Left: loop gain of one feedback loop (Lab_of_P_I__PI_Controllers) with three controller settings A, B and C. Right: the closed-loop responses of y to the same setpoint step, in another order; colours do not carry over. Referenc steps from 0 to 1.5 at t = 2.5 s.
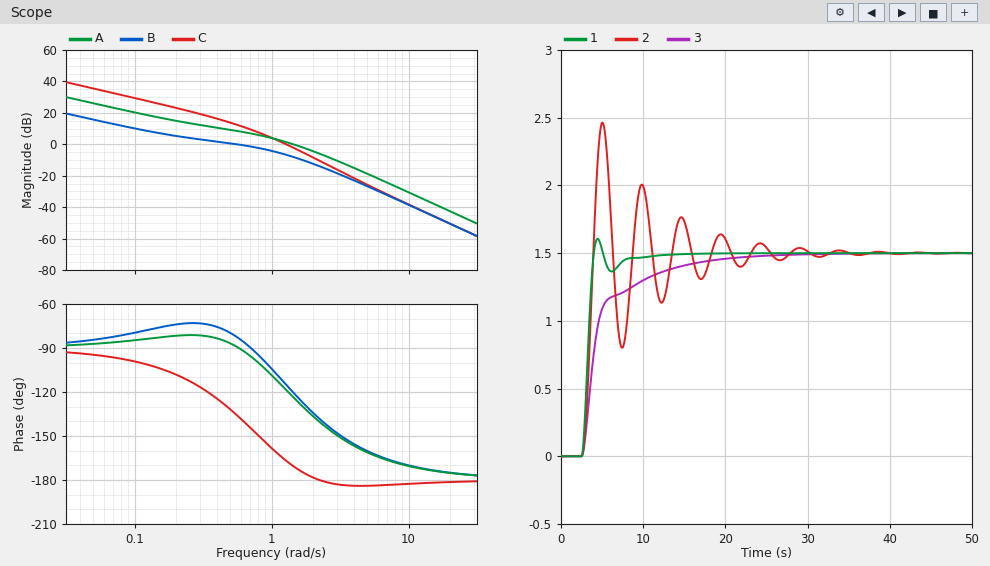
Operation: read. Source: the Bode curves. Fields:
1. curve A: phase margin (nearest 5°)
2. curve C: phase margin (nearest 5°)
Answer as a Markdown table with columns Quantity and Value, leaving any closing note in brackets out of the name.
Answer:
| Quantity | Value |
|---|---|
| curve A: phase margin | 55° |
| curve C: phase margin | 15° |
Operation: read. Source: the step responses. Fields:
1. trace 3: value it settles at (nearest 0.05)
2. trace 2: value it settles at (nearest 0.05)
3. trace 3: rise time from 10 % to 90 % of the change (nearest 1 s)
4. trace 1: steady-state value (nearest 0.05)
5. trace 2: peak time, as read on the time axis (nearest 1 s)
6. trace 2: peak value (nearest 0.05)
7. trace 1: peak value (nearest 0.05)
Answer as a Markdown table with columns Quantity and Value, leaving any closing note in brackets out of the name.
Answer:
| Quantity | Value |
|---|---|
| trace 3: value it settles at | 1.50 |
| trace 2: value it settles at | 1.50 |
| trace 3: rise time from 10 % to 90 % of the change | 9 s |
| trace 1: steady-state value | 1.50 |
| trace 2: peak time, as read on the time axis | 5 s |
| trace 2: peak value | 2.45 |
| trace 1: peak value | 1.60 |
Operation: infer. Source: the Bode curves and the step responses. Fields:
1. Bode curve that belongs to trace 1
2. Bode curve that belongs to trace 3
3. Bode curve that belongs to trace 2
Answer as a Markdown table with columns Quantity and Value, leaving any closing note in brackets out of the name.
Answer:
| Quantity | Value |
|---|---|
| Bode curve that belongs to trace 1 | A |
| Bode curve that belongs to trace 3 | B |
| Bode curve that belongs to trace 2 | C |
